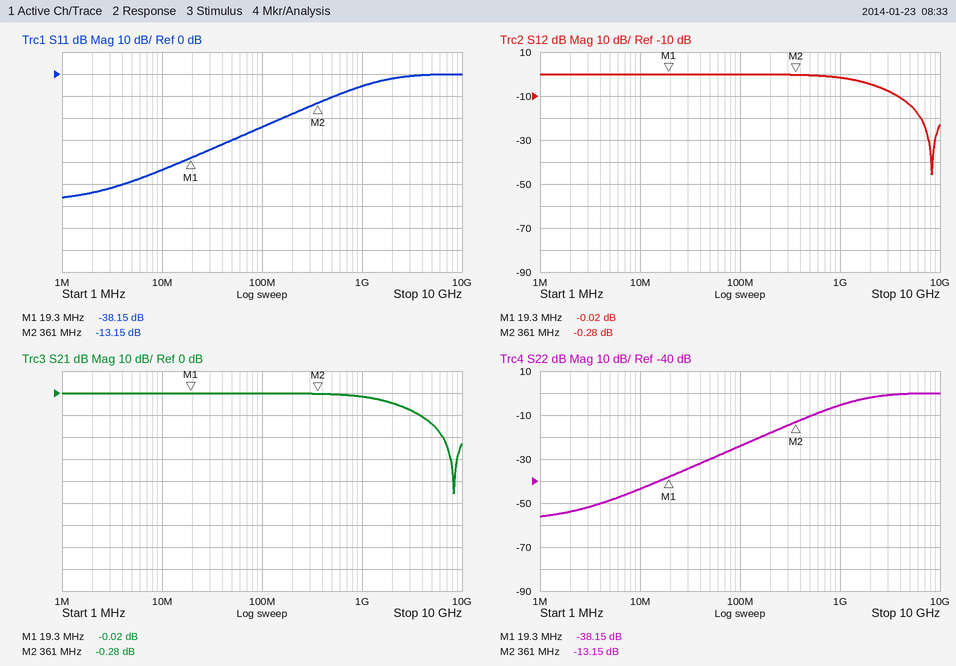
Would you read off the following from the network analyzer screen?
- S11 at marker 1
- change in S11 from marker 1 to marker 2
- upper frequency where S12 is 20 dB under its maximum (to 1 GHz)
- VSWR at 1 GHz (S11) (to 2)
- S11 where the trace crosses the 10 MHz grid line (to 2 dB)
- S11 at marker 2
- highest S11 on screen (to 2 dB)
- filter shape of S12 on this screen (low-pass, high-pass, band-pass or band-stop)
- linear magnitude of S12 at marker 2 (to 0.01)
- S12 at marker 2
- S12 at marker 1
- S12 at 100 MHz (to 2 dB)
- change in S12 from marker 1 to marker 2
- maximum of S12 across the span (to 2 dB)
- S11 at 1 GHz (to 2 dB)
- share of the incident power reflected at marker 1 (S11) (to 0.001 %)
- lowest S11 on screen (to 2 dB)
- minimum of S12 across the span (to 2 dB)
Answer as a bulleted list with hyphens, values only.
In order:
- -38.15 dB
- 25.00 dB
- 6 GHz
- 4
- -44 dB
- -13.15 dB
- 0 dB
- low-pass
- 0.97
- -0.28 dB
- -0.02 dB
- 0 dB
- -0.26 dB
- 0 dB
- -6 dB
- 0.015 %
- -56 dB
- -46 dB
